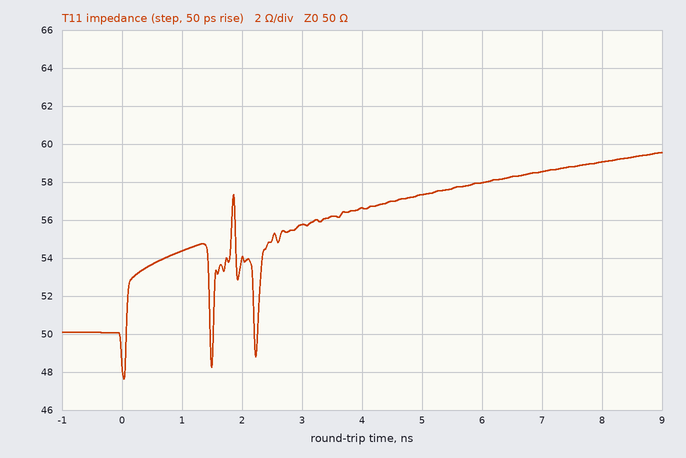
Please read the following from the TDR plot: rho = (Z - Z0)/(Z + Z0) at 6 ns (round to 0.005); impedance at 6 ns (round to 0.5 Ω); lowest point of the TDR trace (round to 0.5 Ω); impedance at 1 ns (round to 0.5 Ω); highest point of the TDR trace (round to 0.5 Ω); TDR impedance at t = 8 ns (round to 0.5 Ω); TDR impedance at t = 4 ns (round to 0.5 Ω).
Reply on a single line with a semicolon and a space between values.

+0.075; 58.0 Ω; 47.5 Ω; 54.5 Ω; 59.5 Ω; 59.0 Ω; 56.5 Ω
